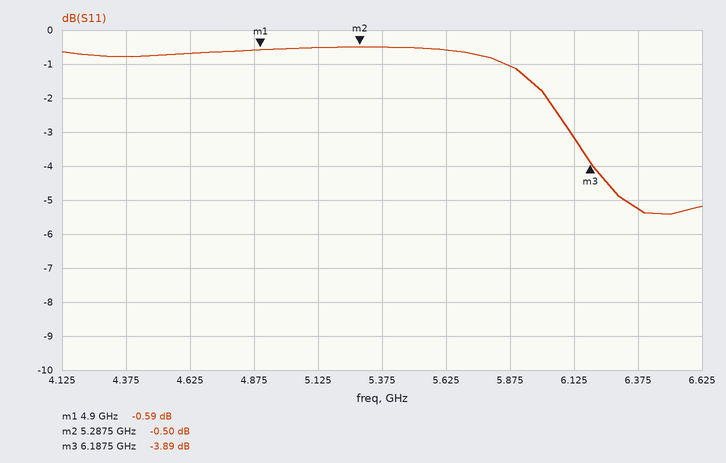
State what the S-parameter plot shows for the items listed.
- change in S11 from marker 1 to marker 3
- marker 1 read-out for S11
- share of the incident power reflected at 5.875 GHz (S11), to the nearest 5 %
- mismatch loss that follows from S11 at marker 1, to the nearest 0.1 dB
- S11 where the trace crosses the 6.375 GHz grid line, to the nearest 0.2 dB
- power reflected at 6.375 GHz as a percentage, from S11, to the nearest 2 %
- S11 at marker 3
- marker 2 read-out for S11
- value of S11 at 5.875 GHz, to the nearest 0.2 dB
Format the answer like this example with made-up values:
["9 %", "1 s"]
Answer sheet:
["-3.30 dB", "-0.59 dB", "80 %", "9.0 dB", "-5.2 dB", "30 %", "-3.89 dB", "-0.50 dB", "-1.0 dB"]
